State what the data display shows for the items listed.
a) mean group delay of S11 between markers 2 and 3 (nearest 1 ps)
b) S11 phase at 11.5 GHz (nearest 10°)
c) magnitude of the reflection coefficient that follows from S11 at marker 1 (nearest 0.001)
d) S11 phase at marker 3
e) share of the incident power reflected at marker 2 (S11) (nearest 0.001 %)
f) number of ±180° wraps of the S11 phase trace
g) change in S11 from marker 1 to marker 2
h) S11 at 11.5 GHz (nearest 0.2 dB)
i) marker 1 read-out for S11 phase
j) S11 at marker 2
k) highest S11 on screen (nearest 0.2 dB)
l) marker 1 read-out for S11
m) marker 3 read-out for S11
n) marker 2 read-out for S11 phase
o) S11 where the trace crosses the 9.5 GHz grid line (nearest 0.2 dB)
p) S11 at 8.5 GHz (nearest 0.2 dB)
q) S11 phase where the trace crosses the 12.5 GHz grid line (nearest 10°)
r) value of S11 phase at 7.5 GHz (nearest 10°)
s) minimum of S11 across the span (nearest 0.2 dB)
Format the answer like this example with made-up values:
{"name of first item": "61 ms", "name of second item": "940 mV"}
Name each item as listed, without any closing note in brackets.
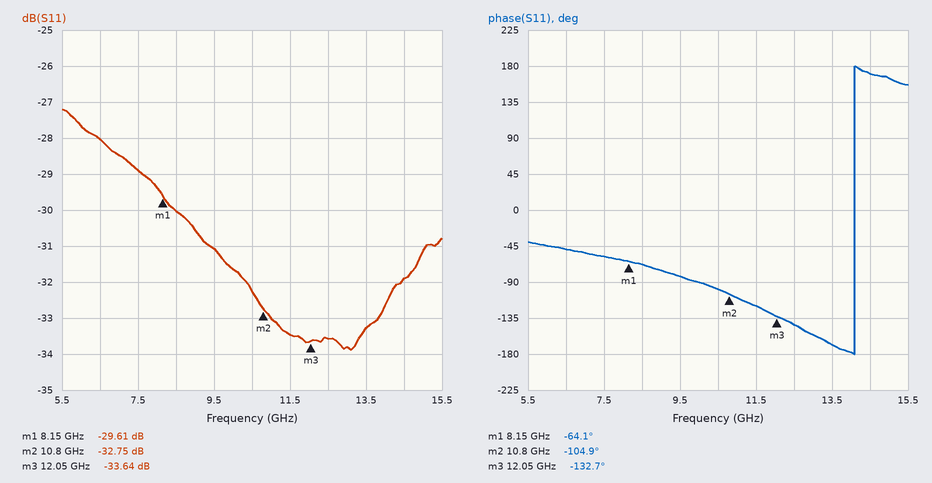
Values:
{"mean group delay of S11 between markers 2 and 3": "62 ps", "S11 phase at 11.5 GHz": "-120°", "magnitude of the reflection coefficient that follows from S11 at marker 1": "0.033", "S11 phase at marker 3": "-132.7°", "share of the incident power reflected at marker 2 (S11)": "0.053 %", "number of ±180° wraps of the S11 phase trace": "1", "change in S11 from marker 1 to marker 2": "-3.14 dB", "S11 at 11.5 GHz": "-33.4 dB", "marker 1 read-out for S11 phase": "-64.1°", "S11 at marker 2": "-32.75 dB", "highest S11 on screen": "-27.2 dB", "marker 1 read-out for S11": "-29.61 dB", "marker 3 read-out for S11": "-33.64 dB", "marker 2 read-out for S11 phase": "-104.9°", "S11 where the trace crosses the 9.5 GHz grid line": "-31.0 dB", "S11 at 8.5 GHz": "-30.0 dB", "S11 phase where the trace crosses the 12.5 GHz grid line": "-140°", "value of S11 phase at 7.5 GHz": "-60°", "minimum of S11 across the span": "-33.8 dB"}
